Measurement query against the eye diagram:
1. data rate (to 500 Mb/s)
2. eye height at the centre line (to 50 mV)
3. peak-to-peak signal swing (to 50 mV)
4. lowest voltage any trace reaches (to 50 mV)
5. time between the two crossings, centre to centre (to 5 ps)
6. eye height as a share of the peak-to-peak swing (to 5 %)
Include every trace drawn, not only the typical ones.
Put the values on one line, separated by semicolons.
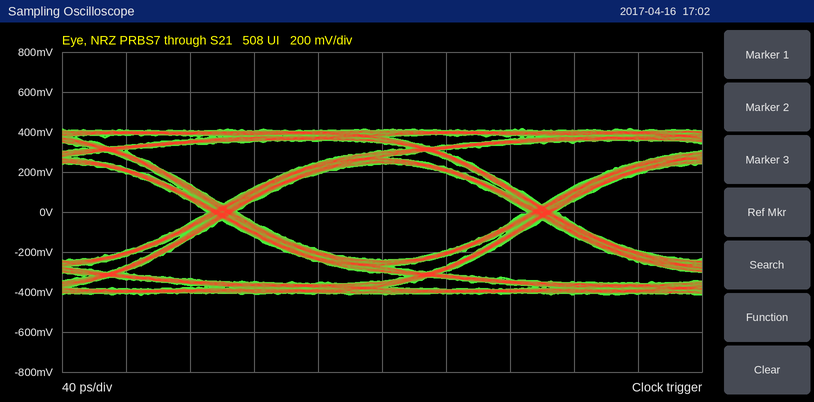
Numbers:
5.0 Gb/s; 500 mV; 850 mV; -400 mV; 200 ps; 60 %
